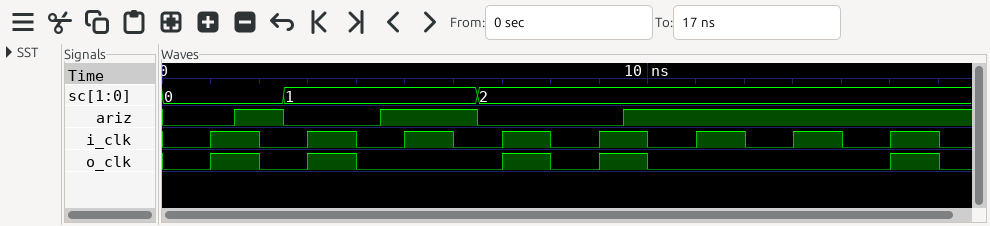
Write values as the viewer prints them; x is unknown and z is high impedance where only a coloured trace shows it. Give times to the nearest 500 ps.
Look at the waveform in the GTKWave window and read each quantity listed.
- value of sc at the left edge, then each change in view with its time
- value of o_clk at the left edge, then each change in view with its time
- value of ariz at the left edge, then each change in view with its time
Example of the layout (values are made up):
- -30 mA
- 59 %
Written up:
- 0, 1 at 2500 ps, 2 at 6500 ps
- 0, 1 at 1000 ps, 0 at 2000 ps, 1 at 3000 ps, 0 at 4000 ps, 1 at 7000 ps, 0 at 8000 ps, 1 at 9000 ps, 0 at 10000 ps, 1 at 15000 ps, 0 at 16000 ps
- 0, 1 at 1500 ps, 0 at 2500 ps, 1 at 4500 ps, 0 at 6500 ps, 1 at 9500 ps
